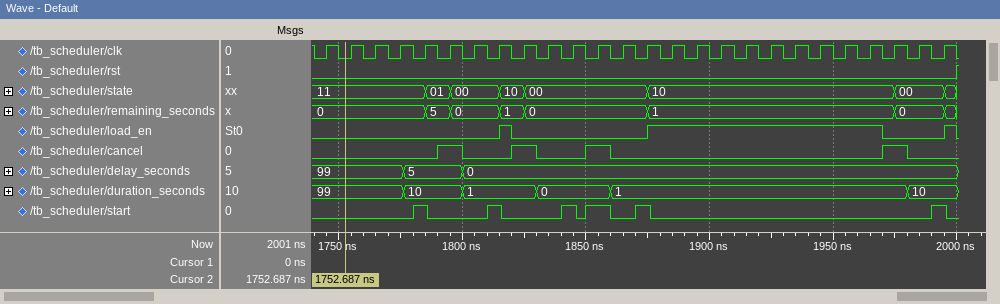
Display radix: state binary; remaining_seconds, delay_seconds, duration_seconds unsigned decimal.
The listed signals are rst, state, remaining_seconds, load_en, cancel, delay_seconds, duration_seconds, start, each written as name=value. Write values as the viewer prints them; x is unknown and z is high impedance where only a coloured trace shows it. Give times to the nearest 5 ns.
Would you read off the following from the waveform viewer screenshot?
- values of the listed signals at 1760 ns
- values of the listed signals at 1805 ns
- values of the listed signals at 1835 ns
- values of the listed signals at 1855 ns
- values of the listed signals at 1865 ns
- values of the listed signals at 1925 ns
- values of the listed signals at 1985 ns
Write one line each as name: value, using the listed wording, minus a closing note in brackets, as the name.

values of the listed signals at 1760 ns: rst=0, state=11, remaining_seconds=0, load_en=0, cancel=0, delay_seconds=99, duration_seconds=99, start=0
values of the listed signals at 1805 ns: rst=0, state=00, remaining_seconds=0, load_en=0, cancel=0, delay_seconds=0, duration_seconds=1, start=0
values of the listed signals at 1835 ns: rst=0, state=00, remaining_seconds=0, load_en=0, cancel=0, delay_seconds=0, duration_seconds=0, start=0
values of the listed signals at 1855 ns: rst=0, state=00, remaining_seconds=0, load_en=0, cancel=1, delay_seconds=0, duration_seconds=0, start=1
values of the listed signals at 1865 ns: rst=0, state=00, remaining_seconds=0, load_en=0, cancel=0, delay_seconds=0, duration_seconds=1, start=0
values of the listed signals at 1925 ns: rst=0, state=10, remaining_seconds=1, load_en=1, cancel=0, delay_seconds=0, duration_seconds=1, start=0
values of the listed signals at 1985 ns: rst=0, state=00, remaining_seconds=0, load_en=0, cancel=0, delay_seconds=0, duration_seconds=10, start=0
